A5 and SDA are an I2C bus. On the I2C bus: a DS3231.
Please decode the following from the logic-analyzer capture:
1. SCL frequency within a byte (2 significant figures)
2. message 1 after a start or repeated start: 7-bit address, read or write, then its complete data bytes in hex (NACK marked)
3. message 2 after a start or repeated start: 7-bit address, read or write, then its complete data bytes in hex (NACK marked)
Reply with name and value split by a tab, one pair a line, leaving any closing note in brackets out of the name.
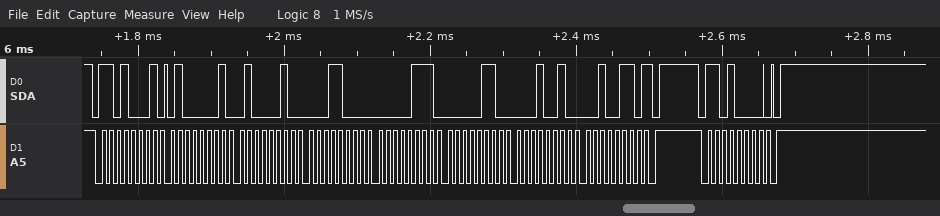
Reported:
SCL frequency within a byte	100 kHz
message 1 after a start or repeated start: 7-bit address, read or write, then its complete data bytes in hex	0x68 read: 41 42 18 07 06 12 26 NACK
message 2 after a start or repeated start: 7-bit address, read or write, then its complete data bytes in hex	0x68 write
